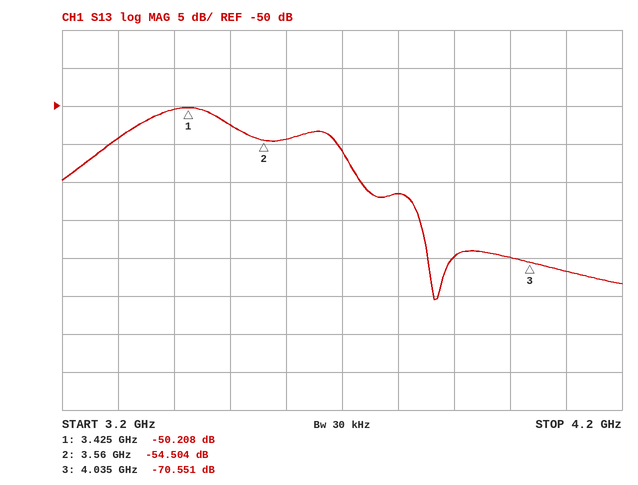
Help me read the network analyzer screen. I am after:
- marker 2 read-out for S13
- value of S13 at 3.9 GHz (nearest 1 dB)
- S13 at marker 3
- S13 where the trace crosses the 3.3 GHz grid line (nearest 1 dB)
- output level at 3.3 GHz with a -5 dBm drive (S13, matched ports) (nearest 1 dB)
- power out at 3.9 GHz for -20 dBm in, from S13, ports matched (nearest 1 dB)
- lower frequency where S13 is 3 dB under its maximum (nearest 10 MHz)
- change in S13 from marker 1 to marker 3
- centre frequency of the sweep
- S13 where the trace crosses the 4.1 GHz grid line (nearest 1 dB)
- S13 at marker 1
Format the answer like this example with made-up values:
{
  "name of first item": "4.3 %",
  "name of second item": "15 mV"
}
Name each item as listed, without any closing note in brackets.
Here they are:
{
  "marker 2 read-out for S13": "-54.504 dB",
  "value of S13 at 3.9 GHz": "-70 dB",
  "S13 at marker 3": "-70.551 dB",
  "S13 where the trace crosses the 3.3 GHz grid line": "-54 dB",
  "output level at 3.3 GHz with a -5 dBm drive (S13, matched ports)": "-59 dBm",
  "power out at 3.9 GHz for -20 dBm in, from S13, ports matched": "-90 dBm",
  "lower frequency where S13 is 3 dB under its maximum": "3.32 GHz",
  "change in S13 from marker 1 to marker 3": "-20.343 dB",
  "centre frequency of the sweep": "3.7 GHz",
  "S13 where the trace crosses the 4.1 GHz grid line": "-72 dB",
  "S13 at marker 1": "-50.208 dB"
}
